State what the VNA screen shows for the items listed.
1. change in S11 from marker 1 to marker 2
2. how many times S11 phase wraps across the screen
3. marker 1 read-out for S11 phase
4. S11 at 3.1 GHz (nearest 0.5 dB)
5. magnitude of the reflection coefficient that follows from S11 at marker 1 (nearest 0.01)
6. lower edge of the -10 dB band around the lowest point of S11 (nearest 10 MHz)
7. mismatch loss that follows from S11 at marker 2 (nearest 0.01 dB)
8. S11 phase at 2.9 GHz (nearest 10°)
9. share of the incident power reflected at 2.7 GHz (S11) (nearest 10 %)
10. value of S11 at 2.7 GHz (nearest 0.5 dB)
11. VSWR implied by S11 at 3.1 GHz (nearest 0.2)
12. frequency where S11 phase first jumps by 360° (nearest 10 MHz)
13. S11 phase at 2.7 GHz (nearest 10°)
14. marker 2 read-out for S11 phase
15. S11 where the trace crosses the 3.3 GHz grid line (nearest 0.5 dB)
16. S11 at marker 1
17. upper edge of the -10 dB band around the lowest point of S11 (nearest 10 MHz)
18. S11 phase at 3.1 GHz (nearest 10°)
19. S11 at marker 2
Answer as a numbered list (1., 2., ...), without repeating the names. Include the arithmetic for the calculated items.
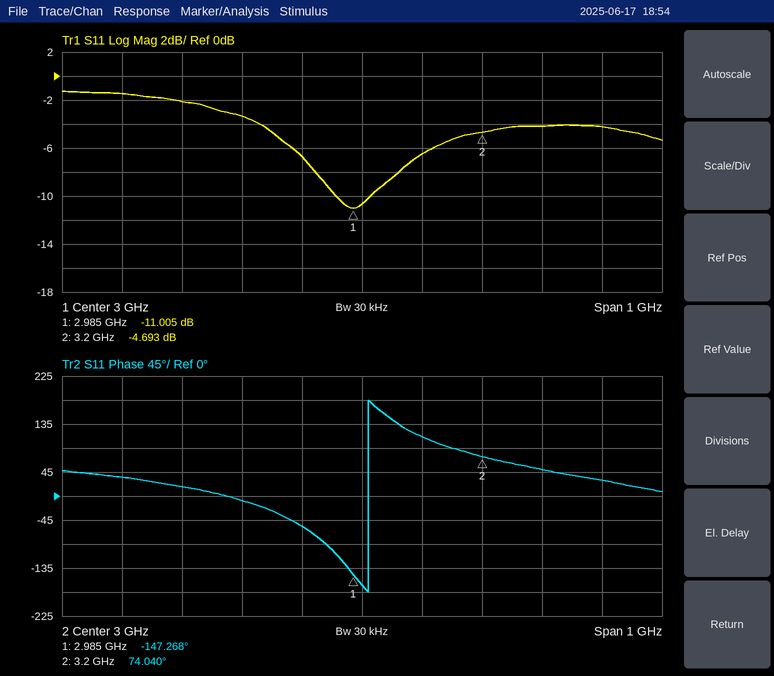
1. -4.693 − (-11.005) = 6.312 dB
2. 1
3. -147.268°
4. -6.5 dB
5. 10^(-11.005/20) ≈ 0.28
6. 2.96 GHz
7. −10 log10(1 − 10^(-4.693/10)) ≈ 1.80 dB
8. -60°
9. 10^(-2/10) ≈ 63.1 %, so 60 % to the nearest 10 %
10. -2.0 dB
11. |Γ| = 10^(-6.5/20) = 0.4732; VSWR = (1 + 0.4732)/(1 − 0.4732) ≈ 2.8
12. 3.01 GHz
13. 20°
14. 74.040°
15. -4.0 dB
16. -11.005 dB
17. 3.01 GHz
18. 110°
19. -4.693 dB
